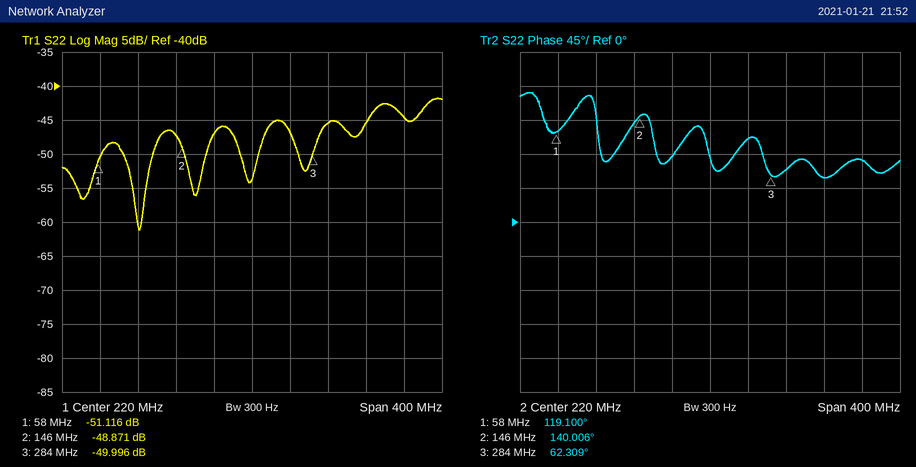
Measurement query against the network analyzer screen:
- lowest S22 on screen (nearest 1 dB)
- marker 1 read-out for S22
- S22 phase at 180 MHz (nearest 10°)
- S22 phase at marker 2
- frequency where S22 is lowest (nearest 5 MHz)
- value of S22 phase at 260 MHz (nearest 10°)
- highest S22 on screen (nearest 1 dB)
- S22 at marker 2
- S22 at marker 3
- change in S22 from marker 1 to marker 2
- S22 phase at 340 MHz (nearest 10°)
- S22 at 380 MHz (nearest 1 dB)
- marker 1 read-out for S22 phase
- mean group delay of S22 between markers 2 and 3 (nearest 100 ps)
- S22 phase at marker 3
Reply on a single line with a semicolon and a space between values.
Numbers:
-61 dB; -51.116 dB; 90°; 140.006°; 100 MHz; 110°; -42 dB; -48.871 dB; -49.996 dB; 2.245 dB; 60°; -45 dB; 119.100°; 1.6 ns; 62.309°
